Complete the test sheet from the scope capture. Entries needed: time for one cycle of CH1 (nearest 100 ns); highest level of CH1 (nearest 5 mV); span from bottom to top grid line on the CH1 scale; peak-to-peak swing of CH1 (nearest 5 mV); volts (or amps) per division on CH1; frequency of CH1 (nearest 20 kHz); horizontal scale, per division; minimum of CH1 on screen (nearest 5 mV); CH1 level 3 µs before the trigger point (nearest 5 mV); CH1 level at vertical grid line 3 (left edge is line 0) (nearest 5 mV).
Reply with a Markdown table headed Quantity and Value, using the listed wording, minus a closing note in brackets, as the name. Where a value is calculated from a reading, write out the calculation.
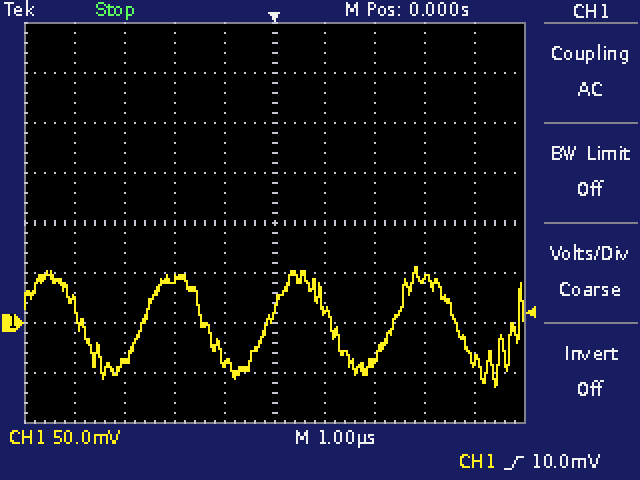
| Quantity | Value |
|---|---|
| time for one cycle of CH1 | 2.5 µs |
| highest level of CH1 | 55 mV |
| span from bottom to top grid line on the CH1 scale | 400 mV |
| peak-to-peak swing of CH1 | 55 mV − (-65 mV) = 120 mV |
| volts (or amps) per division on CH1 | 50 mV |
| frequency of CH1 | 1 / 2.5 µs ≈ 400 kHz |
| horizontal scale, per division | 1 µs |
| minimum of CH1 on screen | -65 mV |
| CH1 level 3 µs before the trigger point | -40 mV |
| CH1 level at vertical grid line 3 (left edge is line 0) | 45 mV |
